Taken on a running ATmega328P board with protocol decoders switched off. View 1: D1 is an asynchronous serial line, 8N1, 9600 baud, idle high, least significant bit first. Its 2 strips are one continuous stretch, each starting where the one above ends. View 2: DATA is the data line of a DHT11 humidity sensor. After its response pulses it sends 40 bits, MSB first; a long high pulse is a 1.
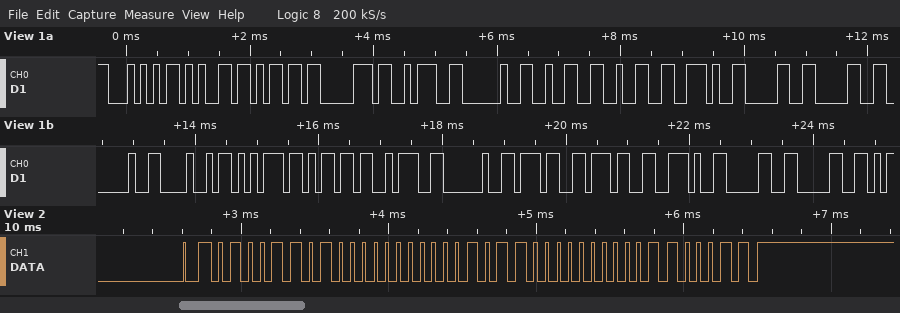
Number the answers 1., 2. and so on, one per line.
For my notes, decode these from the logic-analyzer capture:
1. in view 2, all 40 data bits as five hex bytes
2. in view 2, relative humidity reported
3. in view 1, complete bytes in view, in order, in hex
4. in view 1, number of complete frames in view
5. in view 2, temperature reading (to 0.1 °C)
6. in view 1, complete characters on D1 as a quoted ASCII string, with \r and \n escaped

1. 4D 00 16 00 63
2. 77 %
3. 0x54 0x65 0x6D 0x70 0x3A 0x20 0x32 0x32 0x2E 0x30 0x30 0x20 0x48 0x75 0x6D 0x3A 0x20 0x37 0x37 0x2E 0x30 0x30
4. 22
5. 22.0 °C
6. "Temp: 22.00 Hum: 77.00"
